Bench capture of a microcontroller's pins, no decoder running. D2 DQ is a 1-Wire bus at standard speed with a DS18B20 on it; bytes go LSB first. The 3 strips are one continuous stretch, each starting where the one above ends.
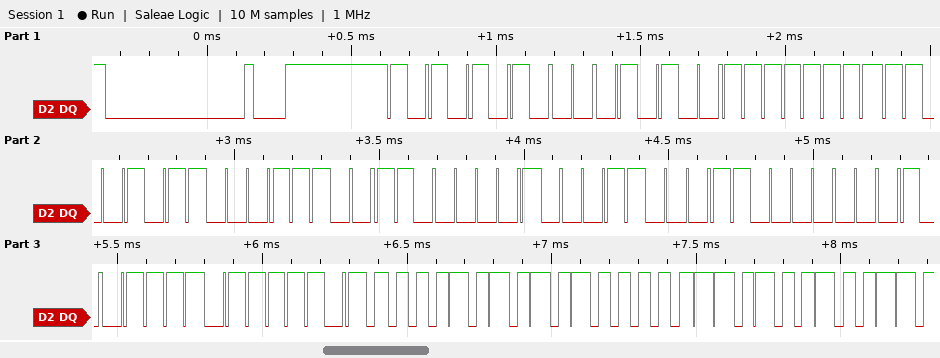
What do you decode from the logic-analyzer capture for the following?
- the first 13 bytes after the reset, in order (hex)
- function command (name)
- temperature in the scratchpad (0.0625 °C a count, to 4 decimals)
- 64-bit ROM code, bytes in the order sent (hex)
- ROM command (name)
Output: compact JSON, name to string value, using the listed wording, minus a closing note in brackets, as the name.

{"the first 13 bytes after the reset, in order": "55 28 FF D3 38 83 18 03 F2 BE 50 05 4B", "function command": "Read Scratchpad", "temperature in the scratchpad": "85.0000 °C", "64-bit ROM code, bytes in the order sent": "28 FF D3 38 83 18 03 F2", "ROM command": "Match ROM"}
